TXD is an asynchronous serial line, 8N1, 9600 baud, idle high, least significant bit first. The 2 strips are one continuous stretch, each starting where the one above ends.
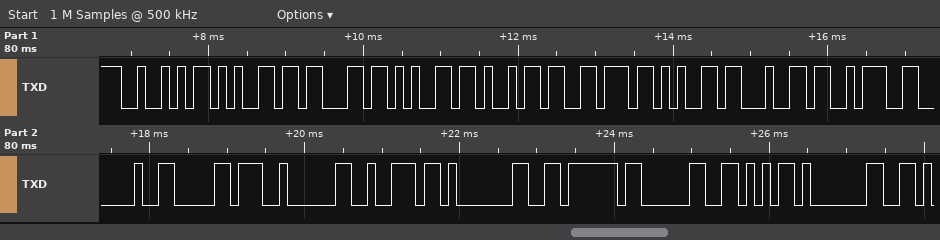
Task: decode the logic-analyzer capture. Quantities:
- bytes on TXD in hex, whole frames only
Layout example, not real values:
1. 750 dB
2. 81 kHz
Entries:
1. 52 65 63 65 69 76 65 64 3A 20 B0 02 72 01 F6 03 56 01
